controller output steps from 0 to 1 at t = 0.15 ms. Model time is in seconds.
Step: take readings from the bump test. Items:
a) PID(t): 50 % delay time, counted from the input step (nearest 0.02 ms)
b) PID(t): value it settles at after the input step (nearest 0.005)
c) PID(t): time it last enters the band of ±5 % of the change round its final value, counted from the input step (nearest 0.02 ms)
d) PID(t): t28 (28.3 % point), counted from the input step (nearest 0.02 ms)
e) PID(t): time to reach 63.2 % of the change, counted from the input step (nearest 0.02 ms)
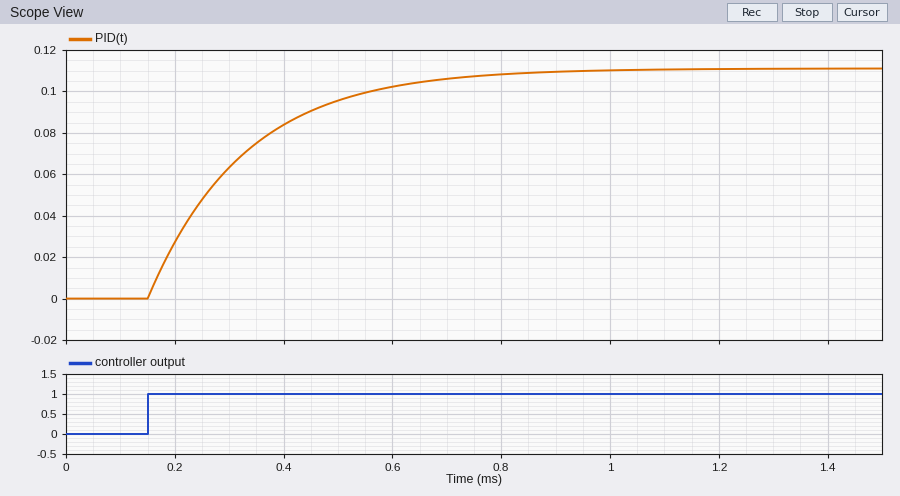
0.12 ms
0.110
0.54 ms
0.06 ms
0.18 ms
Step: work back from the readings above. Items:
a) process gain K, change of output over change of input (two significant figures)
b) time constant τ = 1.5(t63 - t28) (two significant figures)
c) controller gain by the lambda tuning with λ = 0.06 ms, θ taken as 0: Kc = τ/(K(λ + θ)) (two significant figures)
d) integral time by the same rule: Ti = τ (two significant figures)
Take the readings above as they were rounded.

0.11
0.18 ms
27
0.18 ms
